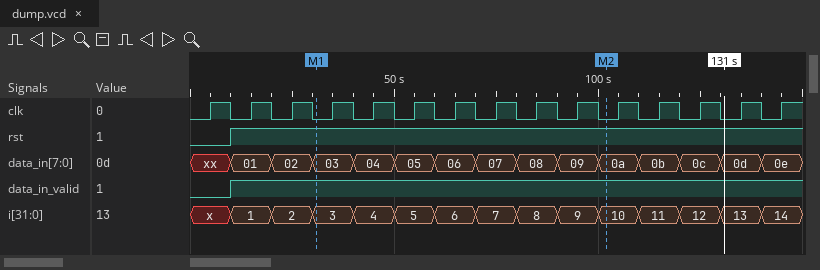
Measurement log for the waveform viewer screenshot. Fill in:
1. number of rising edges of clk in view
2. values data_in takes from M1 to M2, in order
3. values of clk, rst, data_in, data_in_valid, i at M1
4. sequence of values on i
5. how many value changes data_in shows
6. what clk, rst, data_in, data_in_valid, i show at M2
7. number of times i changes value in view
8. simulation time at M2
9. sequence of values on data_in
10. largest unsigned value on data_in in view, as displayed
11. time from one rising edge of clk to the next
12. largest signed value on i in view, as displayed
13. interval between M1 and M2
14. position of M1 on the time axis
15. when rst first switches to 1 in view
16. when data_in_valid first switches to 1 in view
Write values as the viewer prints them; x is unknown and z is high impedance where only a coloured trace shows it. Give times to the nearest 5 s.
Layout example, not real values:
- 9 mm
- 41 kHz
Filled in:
- 15
- 03, 04, 05, 06, 07, 08, 09, 0a
- clk=0, rst=1, data_in=03, data_in_valid=1, i=3
- x, 1, 2, 3, 4, 5, 6, 7, 8, 9, 10, 11, 12, 13, 14
- 14
- clk=0, rst=1, data_in=0a, data_in_valid=1, i=10
- 14
- 100 s
- xx, 01, 02, 03, 04, 05, 06, 07, 08, 09, 0a, 0b, 0c, 0d, 0e
- 0e
- 10 s
- 14
- 70 s
- 30 s
- 10 s
- 10 s
